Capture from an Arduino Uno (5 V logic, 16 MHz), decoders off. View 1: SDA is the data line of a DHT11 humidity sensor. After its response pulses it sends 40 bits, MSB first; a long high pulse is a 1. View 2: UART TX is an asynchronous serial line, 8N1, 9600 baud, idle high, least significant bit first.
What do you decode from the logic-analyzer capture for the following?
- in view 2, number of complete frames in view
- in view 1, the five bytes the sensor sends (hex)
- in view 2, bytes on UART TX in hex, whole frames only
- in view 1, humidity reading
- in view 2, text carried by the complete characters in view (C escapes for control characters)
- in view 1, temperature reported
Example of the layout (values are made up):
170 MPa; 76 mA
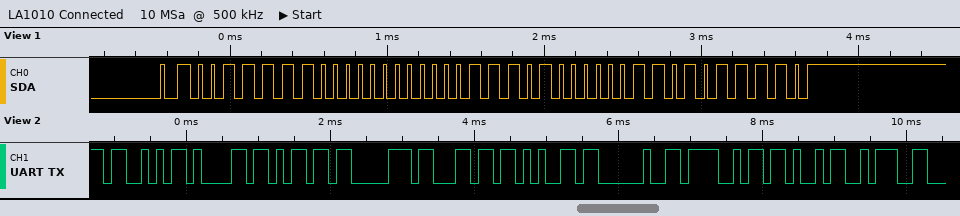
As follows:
10; 3E 00 1D 03 5E; 53 61 6D 70 6C 65 20 4F 4B 3A; 62 %; "Sample OK:"; 29.3 °C
